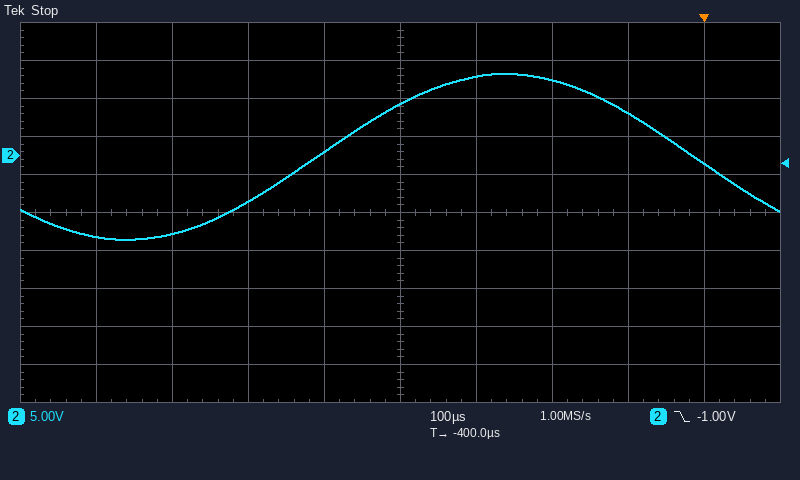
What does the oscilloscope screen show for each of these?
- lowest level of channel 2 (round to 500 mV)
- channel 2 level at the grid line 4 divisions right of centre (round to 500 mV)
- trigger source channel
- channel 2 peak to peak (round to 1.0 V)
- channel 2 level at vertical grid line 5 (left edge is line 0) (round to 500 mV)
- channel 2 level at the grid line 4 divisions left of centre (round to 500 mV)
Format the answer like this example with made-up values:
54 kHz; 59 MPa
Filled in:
-11.0 V; -1.0 V; channel 2; 22.0 V; 7.0 V; -10.5 V
